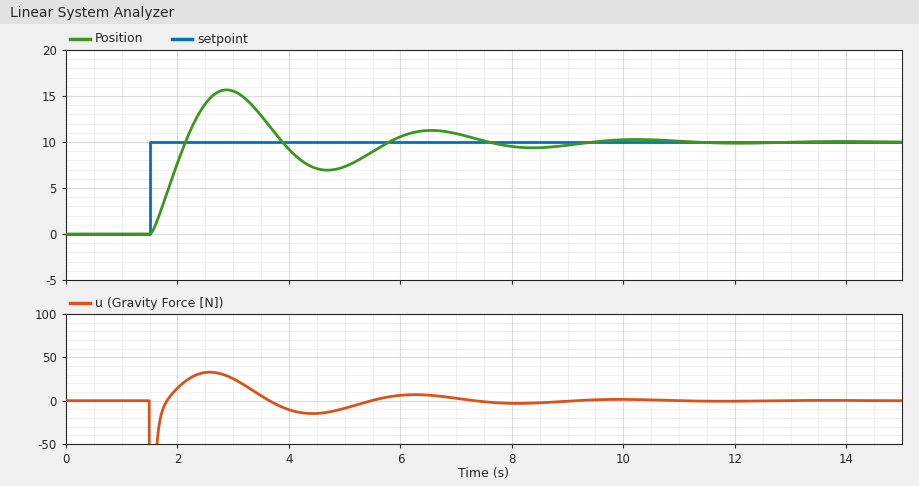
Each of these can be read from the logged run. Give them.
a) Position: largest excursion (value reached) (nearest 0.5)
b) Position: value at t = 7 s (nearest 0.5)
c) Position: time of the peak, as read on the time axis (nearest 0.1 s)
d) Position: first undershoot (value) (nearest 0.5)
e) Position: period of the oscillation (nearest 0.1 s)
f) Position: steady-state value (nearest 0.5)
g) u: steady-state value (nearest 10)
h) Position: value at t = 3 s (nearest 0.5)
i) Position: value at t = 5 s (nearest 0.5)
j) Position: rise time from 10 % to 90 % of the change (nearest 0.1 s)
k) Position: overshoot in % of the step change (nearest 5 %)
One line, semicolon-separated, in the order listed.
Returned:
15.5; 11.0; 2.9 s; 7.0; 3.7 s; 10.0; 0; 15.5; 7.5; 0.5 s; 55 %
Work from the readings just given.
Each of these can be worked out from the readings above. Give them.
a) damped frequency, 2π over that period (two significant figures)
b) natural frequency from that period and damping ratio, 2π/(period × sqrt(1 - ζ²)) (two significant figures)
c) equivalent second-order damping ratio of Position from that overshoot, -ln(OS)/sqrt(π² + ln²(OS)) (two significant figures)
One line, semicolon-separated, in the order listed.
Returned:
1.7 rad/s; 1.7 rad/s; 0.19
